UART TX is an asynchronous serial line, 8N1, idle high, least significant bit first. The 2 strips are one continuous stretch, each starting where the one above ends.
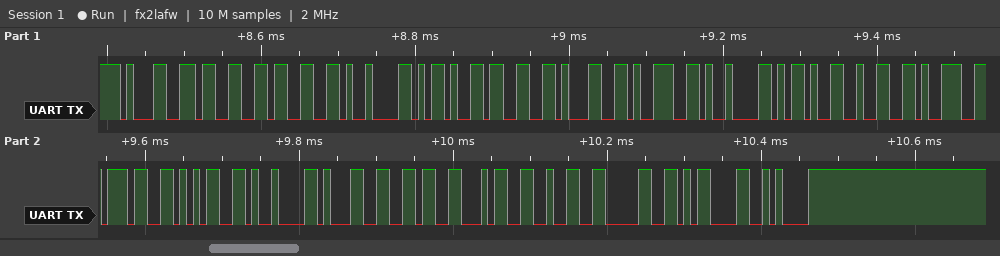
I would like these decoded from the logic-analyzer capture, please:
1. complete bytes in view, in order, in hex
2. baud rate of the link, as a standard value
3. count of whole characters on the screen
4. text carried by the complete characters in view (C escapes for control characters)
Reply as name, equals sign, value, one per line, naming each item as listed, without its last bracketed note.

complete bytes in view, in order, in hex = 31 33 33 09 2D 33 31 39 09 2D 32 39 37 35 09 31 36 34 32 30 0D 0A
baud rate of the link, as a standard value = 115200 baud
count of whole characters on the screen = 22
text carried by the complete characters in view = "133\t-319\t-2975\t16420\r\n"
